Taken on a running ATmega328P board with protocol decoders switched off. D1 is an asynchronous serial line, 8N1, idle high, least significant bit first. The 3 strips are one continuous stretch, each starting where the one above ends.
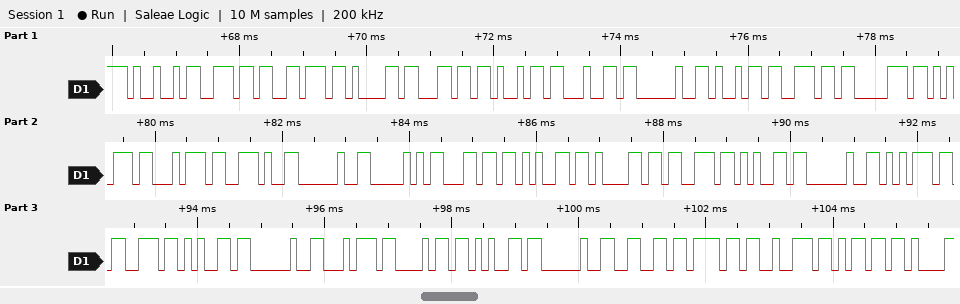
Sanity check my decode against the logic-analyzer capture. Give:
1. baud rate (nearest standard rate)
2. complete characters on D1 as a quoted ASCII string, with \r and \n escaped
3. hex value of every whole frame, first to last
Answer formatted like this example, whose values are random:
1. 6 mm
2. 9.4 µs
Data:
1. 9600 baud
2. "Invalid input. Please use the form"
3. 49 6E 76 61 6C 69 64 20 69 6E 70 75 74 2E 20 50 6C 65 61 73 65 20 75 73 65 20 74 68 65 20 66 6F 72 6D
